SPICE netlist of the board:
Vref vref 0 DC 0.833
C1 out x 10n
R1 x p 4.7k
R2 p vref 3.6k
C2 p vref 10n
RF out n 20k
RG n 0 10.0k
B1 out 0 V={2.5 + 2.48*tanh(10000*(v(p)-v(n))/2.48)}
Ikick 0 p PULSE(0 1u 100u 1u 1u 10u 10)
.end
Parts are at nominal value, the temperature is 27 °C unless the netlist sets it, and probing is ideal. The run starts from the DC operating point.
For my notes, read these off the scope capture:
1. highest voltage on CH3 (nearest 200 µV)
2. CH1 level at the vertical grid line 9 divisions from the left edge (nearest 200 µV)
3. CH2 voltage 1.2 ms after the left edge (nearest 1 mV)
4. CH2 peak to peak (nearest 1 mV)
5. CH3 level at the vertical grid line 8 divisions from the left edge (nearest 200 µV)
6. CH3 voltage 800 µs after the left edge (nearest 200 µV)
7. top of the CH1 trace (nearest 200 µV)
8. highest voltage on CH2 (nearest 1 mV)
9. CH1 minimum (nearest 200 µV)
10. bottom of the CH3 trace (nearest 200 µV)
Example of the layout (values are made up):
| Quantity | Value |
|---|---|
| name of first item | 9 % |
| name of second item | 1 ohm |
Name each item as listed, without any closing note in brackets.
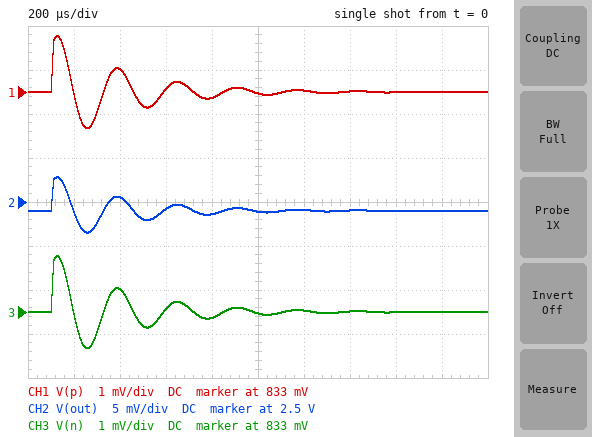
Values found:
| Quantity | Value |
|---|---|
| highest voltage on CH3 | 834.2 mV |
| CH1 level at the vertical grid line 9 divisions from the left edge | 833.0 mV |
| CH2 voltage 1.2 ms after the left edge | 2.499 V |
| CH2 peak to peak | 6 mV |
| CH3 level at the vertical grid line 8 divisions from the left edge | 833.0 mV |
| CH3 voltage 800 µs after the left edge | 832.8 mV |
| top of the CH1 trace | 834.2 mV |
| highest voltage on CH2 | 2.503 V |
| CH1 minimum | 832.2 mV |
| bottom of the CH3 trace | 832.2 mV |
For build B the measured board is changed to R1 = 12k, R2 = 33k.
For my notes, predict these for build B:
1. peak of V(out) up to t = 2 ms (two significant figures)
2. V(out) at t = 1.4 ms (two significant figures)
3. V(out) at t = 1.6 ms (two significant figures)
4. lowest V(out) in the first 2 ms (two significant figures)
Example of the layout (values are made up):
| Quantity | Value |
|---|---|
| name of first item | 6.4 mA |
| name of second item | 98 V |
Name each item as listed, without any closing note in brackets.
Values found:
| Quantity | Value |
|---|---|
| peak of V(out) up to t = 2 ms | 3.6 V |
| V(out) at t = 1.4 ms | 2.4 V |
| V(out) at t = 1.6 ms | 2.7 V |
| lowest V(out) in the first 2 ms | 2.3 V |
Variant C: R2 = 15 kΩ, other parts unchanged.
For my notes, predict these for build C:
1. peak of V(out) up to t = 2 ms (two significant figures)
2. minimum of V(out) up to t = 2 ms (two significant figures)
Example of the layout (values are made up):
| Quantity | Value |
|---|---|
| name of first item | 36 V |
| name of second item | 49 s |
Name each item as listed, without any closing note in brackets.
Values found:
| Quantity | Value |
|---|---|
| peak of V(out) up to t = 2 ms | 5.0 V |
| minimum of V(out) up to t = 2 ms | 20 mV |
